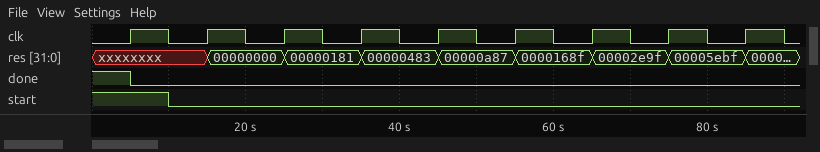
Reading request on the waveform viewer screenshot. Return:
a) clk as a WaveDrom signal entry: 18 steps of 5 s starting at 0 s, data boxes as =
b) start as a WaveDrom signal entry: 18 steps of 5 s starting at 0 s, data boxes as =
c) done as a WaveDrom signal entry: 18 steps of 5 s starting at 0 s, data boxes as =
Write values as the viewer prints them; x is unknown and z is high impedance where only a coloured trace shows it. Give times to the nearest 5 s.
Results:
{name: 'clk', wave: '010101010101010101'}
{name: 'start', wave: '1.0...............'}
{name: 'done', wave: '10................'}
